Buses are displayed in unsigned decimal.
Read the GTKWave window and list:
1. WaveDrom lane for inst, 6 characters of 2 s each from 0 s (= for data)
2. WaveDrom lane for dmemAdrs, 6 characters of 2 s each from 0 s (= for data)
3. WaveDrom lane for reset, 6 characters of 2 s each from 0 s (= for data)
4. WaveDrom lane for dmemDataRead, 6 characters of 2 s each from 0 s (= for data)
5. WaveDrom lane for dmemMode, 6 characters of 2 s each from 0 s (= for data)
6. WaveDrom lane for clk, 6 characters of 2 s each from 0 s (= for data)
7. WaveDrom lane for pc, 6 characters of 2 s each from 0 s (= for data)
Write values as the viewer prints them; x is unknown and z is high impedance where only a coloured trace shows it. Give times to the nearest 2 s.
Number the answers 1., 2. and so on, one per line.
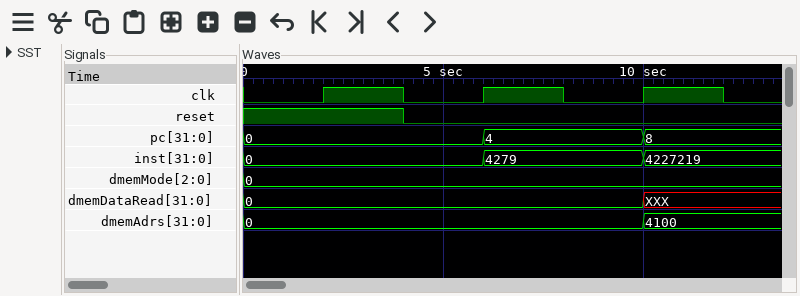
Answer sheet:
1. {name: 'inst', wave: '=..=.=', data: '0 4279 4227219'}
2. {name: 'dmemAdrs', wave: '=....=', data: '0 4100'}
3. {name: 'reset', wave: '1.0...'}
4. {name: 'dmemDataRead', wave: '=....x', data: '0'}
5. {name: 'dmemMode', wave: '=.....', data: '0'}
6. {name: 'clk', wave: '010101'}
7. {name: 'pc', wave: '=..=.=', data: '0 4 8'}
